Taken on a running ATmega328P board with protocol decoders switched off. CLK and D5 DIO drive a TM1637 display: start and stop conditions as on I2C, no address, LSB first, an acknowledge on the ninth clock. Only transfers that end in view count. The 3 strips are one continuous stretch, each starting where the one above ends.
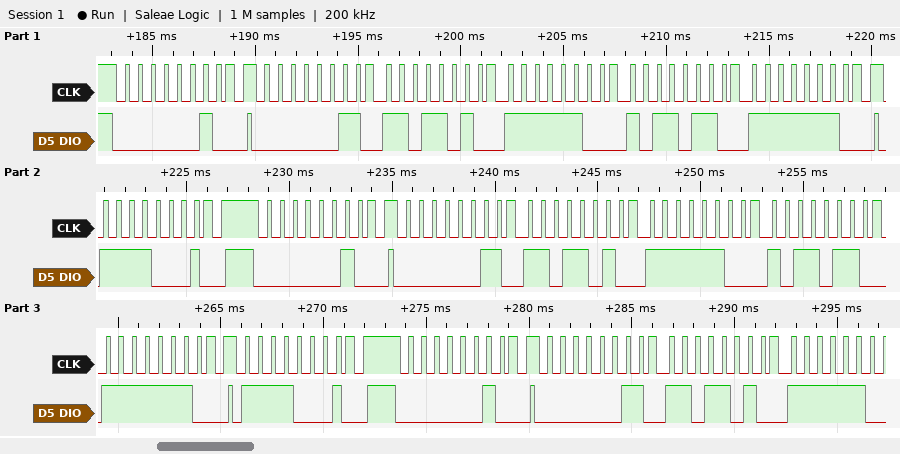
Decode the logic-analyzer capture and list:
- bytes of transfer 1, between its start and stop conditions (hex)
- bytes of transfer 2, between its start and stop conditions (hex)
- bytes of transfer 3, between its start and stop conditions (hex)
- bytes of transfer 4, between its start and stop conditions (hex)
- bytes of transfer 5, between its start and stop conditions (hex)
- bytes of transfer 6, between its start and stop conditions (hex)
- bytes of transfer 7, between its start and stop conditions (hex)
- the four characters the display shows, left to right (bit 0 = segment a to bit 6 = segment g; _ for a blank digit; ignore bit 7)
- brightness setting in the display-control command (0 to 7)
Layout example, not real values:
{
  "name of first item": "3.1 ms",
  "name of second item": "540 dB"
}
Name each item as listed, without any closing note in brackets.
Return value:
{
  "bytes of transfer 1, between its start and stop conditions": "40",
  "bytes of transfer 2, between its start and stop conditions": "C0 5B 3F 6D 7F",
  "bytes of transfer 3, between its start and stop conditions": "8F",
  "bytes of transfer 4, between its start and stop conditions": "40",
  "bytes of transfer 5, between its start and stop conditions": "C0 5B 3F 6D 7F",
  "bytes of transfer 6, between its start and stop conditions": "8F",
  "bytes of transfer 7, between its start and stop conditions": "40",
  "the four characters the display shows, left to right": "2058",
  "brightness setting in the display-control command": "7"
}
